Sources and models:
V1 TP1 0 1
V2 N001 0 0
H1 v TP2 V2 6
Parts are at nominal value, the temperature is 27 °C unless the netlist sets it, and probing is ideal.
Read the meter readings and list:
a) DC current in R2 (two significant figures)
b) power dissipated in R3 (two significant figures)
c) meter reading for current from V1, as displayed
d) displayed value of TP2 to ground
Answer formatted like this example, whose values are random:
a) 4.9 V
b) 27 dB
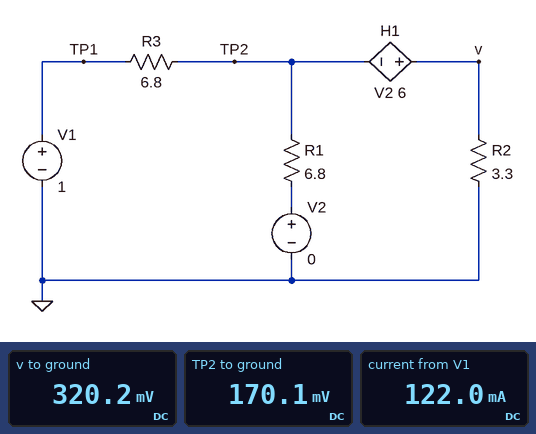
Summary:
a) 97 mA
b) 100 mW
c) 122.0 mA
d) 170.1 mV
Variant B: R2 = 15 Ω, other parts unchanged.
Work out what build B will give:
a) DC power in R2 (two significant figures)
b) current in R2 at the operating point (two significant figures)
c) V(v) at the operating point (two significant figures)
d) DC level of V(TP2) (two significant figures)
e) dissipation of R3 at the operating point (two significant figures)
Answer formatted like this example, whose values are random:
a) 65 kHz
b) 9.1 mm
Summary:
a) 29 mW
b) 44 mA
c) 660 mV
d) 350 mV
e) 62 mW
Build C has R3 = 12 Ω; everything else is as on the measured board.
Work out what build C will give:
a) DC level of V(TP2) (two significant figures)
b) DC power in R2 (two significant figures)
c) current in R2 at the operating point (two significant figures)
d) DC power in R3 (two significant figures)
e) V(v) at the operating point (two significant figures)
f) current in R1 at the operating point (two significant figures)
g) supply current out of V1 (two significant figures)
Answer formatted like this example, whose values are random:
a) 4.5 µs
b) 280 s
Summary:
a) 100 mV
b) 12 mW
c) 59 mA
d) 67 mW
e) 200 mV
f) 15 mA
g) 75 mA
